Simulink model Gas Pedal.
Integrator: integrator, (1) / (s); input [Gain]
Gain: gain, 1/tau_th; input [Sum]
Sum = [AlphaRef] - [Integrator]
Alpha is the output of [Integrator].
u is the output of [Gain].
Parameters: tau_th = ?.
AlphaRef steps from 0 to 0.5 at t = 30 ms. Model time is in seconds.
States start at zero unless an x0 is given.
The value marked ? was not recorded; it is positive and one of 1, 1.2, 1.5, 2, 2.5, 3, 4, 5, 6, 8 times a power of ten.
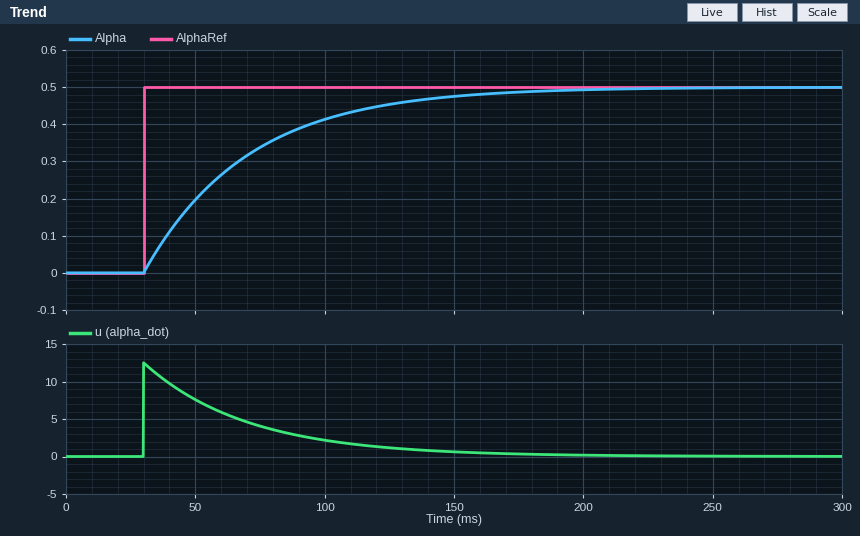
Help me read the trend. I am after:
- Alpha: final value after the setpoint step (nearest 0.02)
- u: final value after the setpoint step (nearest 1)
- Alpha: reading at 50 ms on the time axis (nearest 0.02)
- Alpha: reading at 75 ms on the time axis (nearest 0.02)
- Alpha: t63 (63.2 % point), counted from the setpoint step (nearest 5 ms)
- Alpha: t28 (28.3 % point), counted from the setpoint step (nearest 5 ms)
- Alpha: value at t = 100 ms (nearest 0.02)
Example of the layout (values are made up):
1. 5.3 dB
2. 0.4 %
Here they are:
1. 0.50
2. 0
3. 0.20
4. 0.34
5. 40 ms
6. 15 ms
7. 0.42
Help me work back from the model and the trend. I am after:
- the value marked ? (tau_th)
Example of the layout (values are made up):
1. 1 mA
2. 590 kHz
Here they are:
1. 0.04
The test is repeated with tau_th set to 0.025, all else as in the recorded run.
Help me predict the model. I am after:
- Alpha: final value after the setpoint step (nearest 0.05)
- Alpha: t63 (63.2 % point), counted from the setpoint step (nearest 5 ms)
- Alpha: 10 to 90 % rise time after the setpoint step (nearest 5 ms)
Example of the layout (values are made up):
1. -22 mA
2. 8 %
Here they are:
1. 0.50
2. 25 ms
3. 55 ms
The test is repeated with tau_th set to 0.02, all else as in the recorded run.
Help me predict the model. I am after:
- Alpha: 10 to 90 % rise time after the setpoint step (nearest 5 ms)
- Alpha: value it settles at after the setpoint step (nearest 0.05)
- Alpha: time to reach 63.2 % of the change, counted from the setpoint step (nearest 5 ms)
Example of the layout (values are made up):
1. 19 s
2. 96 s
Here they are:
1. 45 ms
2. 0.50
3. 20 ms
